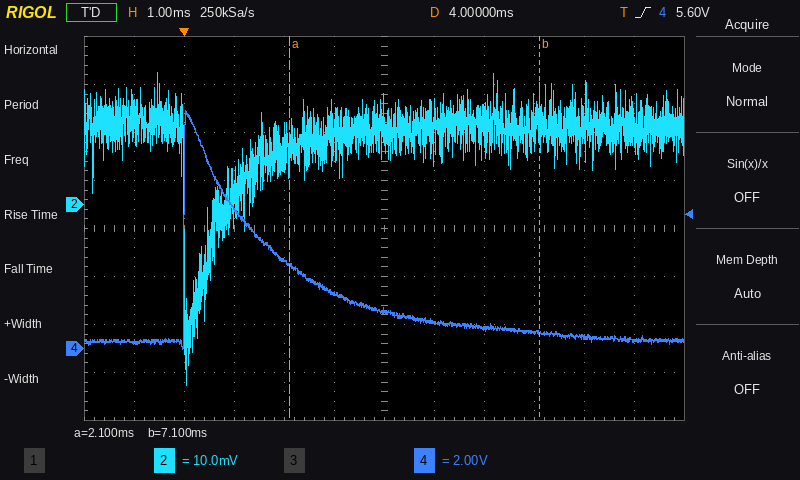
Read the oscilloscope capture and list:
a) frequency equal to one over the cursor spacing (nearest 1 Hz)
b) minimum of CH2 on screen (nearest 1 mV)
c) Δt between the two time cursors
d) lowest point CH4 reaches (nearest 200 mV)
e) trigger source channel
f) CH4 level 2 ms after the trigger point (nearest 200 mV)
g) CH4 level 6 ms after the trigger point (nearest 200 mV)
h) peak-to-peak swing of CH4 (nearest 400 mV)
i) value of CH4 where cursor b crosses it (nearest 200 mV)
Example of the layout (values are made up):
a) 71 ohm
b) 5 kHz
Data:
a) 200 Hz
b) -38 mV
c) 5.0 ms
d) 0.0 V
e) CH4
f) 3.6 V
g) 800 mV
h) 10.0 V
i) 600 mV
